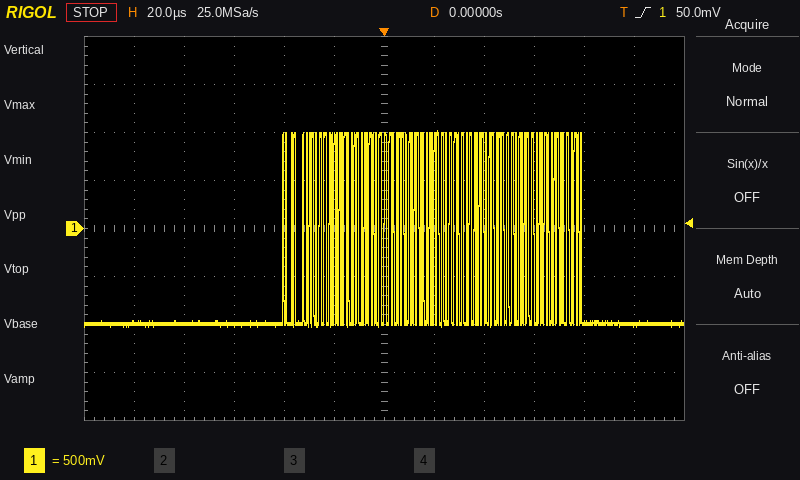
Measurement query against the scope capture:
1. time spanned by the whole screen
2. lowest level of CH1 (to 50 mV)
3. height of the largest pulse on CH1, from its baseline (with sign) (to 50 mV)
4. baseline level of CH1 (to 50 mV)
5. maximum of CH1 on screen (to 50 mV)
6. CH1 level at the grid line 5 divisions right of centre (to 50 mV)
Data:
240 µs
-1.00 V
+2.00 V
-1.00 V
1.00 V
-1.00 V
